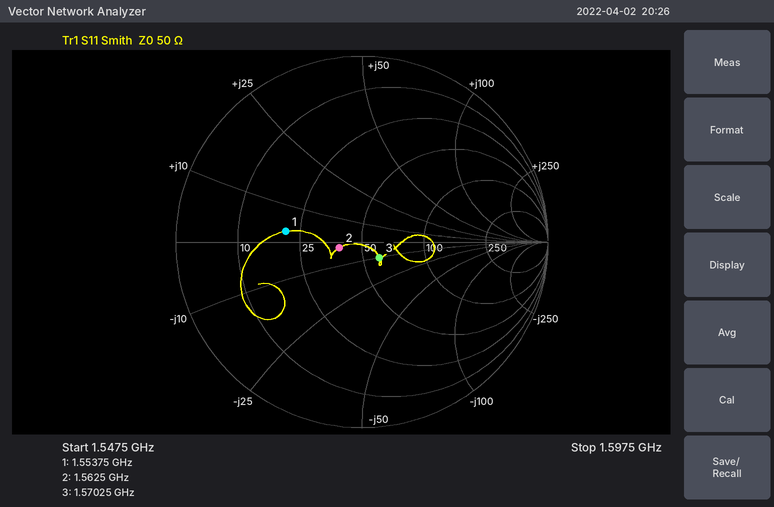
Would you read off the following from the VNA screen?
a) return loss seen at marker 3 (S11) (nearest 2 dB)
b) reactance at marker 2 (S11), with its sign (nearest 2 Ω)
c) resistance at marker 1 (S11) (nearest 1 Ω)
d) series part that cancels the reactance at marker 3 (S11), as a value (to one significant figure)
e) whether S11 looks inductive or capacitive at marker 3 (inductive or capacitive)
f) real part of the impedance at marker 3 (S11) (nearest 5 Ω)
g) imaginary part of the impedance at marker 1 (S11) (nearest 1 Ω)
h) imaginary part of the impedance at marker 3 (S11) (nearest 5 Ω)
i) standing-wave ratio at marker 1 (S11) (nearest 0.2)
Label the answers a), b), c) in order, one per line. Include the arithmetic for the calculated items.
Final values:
a) 18 dB
b) -2 Ω
c) 21 Ω
d) L = 10 Ω/(2π × 1.57025 GHz) ≈ 1 nH
e) capacitive
f) 60 Ω
g) +3 Ω
h) -10 Ω
i) 2.4
